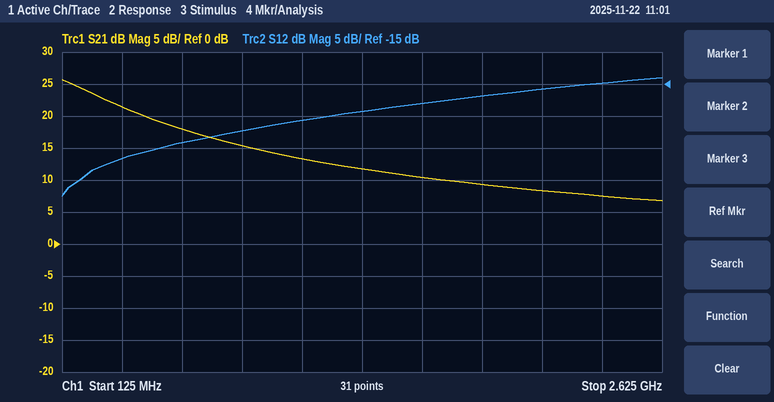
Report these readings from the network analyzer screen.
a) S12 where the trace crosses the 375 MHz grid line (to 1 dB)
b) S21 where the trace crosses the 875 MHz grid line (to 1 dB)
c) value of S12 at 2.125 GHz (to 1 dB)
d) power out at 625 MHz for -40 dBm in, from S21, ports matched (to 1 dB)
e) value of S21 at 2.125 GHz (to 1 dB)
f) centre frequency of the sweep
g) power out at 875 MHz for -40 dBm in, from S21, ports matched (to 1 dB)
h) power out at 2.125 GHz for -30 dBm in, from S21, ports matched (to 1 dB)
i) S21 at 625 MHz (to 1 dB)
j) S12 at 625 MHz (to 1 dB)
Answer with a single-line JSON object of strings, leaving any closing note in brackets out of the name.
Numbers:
{"S12 where the trace crosses the 375 MHz grid line": "-27 dB", "S21 where the trace crosses the 875 MHz grid line": "15 dB", "value of S12 at 2.125 GHz": "-16 dB", "power out at 625 MHz for -40 dBm in, from S21, ports matched": "-22 dBm", "value of S21 at 2.125 GHz": "8 dB", "centre frequency of the sweep": "1.375 GHz", "power out at 875 MHz for -40 dBm in, from S21, ports matched": "-25 dBm", "power out at 2.125 GHz for -30 dBm in, from S21, ports matched": "-22 dBm", "S21 at 625 MHz": "18 dB", "S12 at 625 MHz": "-24 dB"}
